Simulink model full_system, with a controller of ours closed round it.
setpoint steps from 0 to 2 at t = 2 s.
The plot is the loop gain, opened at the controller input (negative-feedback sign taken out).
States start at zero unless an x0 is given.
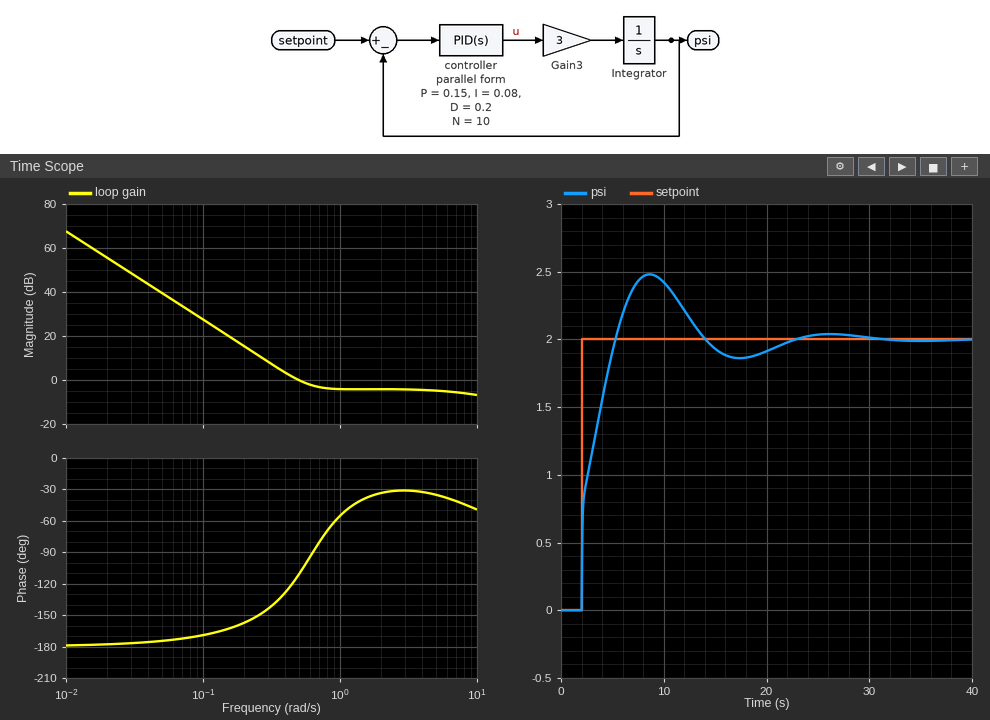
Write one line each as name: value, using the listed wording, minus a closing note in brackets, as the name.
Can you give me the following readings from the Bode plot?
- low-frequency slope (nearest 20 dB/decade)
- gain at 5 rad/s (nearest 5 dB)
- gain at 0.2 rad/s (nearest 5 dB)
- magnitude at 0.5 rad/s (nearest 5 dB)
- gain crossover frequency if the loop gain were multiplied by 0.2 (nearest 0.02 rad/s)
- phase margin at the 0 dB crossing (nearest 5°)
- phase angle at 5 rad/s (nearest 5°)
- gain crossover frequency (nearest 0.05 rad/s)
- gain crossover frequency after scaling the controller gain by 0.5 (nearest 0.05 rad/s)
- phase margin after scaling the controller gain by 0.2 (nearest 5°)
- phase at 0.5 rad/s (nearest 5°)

low-frequency slope: -40 dB/decade
gain at 5 rad/s: -5 dB
gain at 0.2 rad/s: 15 dB
magnitude at 0.5 rad/s: 0 dB
gain crossover frequency if the loop gain were multiplied by 0.2: 0.22 rad/s
phase margin at the 0 dB crossing: 70°
phase angle at 5 rad/s: -35°
gain crossover frequency: 0.50 rad/s
gain crossover frequency after scaling the controller gain by 0.5: 0.35 rad/s
phase margin after scaling the controller gain by 0.2: 25°
phase at 0.5 rad/s: -110°
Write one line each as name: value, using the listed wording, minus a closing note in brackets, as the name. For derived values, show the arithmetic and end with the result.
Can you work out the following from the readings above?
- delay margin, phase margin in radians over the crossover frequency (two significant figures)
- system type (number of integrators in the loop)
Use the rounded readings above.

delay margin, phase margin in radians over the crossover frequency: 70 × π / 180 / 0.5 = 2.4 s
system type: 2
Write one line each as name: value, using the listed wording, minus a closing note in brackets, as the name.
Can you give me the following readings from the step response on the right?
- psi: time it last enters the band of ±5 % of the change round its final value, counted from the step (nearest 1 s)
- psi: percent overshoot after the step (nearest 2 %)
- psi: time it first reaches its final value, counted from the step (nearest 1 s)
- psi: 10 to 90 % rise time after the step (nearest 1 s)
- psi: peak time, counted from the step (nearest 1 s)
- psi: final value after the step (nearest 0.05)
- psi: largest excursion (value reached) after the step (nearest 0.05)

psi: time it last enters the band of ±5 % of the change round its final value, counted from the step: 18 s
psi: percent overshoot after the step: 24 %
psi: time it first reaches its final value, counted from the step: 3 s
psi: 10 to 90 % rise time after the step: 3 s
psi: peak time, counted from the step: 7 s
psi: final value after the step: 2.00
psi: largest excursion (value reached) after the step: 2.50
